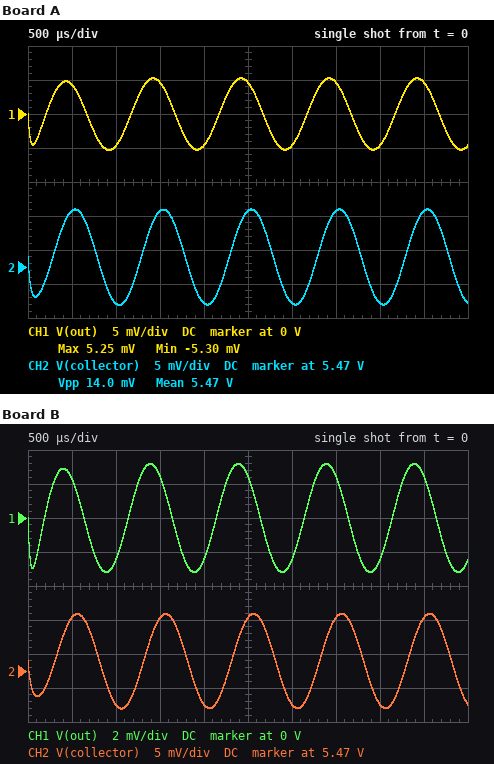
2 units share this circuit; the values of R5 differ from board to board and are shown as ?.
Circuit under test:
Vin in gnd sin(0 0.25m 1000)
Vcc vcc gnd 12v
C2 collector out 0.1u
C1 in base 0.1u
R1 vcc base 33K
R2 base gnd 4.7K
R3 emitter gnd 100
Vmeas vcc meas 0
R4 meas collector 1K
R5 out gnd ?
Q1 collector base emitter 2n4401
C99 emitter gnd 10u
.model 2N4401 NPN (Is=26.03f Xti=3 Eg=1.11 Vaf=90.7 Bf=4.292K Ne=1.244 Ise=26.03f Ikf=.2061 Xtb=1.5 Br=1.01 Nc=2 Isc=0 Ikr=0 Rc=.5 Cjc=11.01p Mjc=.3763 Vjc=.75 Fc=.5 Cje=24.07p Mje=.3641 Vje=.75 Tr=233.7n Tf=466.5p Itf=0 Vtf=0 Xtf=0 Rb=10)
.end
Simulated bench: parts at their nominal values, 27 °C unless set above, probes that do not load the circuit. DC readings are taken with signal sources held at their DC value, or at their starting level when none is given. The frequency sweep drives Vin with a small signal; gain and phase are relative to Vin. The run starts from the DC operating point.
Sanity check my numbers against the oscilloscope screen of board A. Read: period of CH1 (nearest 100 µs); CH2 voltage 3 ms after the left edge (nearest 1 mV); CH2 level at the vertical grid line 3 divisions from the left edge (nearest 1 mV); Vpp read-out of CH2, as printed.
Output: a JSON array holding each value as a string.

["1.0 ms", "5.465 V", "5.478 V", "14.0 mV"]
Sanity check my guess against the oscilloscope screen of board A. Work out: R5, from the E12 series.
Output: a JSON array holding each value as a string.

["1.8 kΩ"]
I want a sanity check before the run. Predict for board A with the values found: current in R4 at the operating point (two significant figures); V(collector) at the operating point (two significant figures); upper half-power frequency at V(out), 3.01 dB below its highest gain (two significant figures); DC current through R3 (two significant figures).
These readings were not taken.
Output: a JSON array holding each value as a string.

["6.5 mA", "5.5 V", "13 MHz", "6.6 mA"]
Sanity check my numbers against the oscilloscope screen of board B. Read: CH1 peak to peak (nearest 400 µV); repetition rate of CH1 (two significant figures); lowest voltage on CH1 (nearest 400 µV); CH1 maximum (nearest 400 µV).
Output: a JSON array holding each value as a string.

["6.4 mV", "1.0 kHz", "-3.2 mV", "3.2 mV"]
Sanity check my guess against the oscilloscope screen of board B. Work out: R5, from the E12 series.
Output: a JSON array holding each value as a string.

["820 Ω"]
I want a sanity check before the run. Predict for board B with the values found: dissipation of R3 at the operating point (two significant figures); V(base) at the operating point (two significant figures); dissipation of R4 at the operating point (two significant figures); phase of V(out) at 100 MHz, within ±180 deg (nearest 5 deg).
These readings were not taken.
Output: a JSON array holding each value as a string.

["4.3 mW", "1.3 V", "43 mW", "85 deg"]
